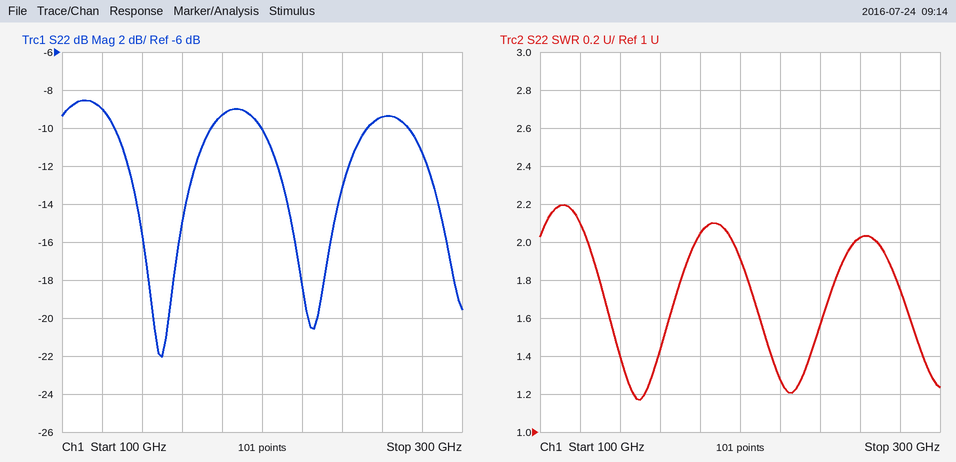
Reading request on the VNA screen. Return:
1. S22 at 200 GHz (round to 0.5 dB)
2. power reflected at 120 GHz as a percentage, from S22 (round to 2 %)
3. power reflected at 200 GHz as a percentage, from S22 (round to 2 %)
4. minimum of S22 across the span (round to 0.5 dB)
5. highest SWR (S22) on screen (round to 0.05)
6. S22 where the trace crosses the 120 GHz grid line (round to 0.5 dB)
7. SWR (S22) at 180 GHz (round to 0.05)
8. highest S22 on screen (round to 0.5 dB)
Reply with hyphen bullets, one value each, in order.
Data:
- -10.0 dB
- 12 %
- 10 %
- -22.0 dB
- 2.20
- -9.0 dB
- 2.05
- -8.5 dB
